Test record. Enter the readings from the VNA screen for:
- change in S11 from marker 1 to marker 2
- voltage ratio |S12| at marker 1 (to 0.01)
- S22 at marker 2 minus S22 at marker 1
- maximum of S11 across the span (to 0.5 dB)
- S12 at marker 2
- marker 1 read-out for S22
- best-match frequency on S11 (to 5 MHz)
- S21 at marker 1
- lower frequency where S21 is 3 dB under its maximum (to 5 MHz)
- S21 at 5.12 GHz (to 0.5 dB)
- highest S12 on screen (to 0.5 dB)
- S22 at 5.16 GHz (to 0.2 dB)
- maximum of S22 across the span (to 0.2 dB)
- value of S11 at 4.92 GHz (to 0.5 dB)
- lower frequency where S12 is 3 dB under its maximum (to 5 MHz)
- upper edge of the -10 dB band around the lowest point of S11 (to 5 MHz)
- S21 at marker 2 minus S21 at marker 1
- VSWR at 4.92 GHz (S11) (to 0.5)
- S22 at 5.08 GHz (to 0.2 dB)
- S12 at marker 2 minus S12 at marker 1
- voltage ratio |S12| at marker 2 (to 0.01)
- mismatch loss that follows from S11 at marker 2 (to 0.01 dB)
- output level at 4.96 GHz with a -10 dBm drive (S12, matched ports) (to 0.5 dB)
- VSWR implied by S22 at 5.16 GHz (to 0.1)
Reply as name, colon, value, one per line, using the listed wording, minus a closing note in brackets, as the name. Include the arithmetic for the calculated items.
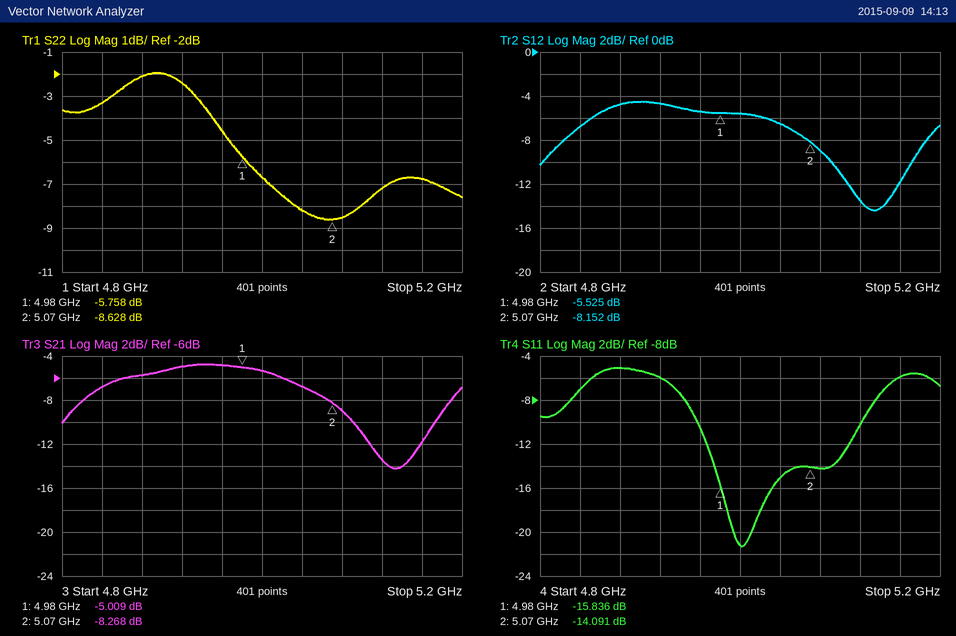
change in S11 from marker 1 to marker 2: -14.091 − (-15.836) = 1.745 dB
voltage ratio |S12| at marker 1: 10^(-5.525/20) ≈ 0.53
S22 at marker 2 minus S22 at marker 1: -8.628 − (-5.758) = -2.870 dB
maximum of S11 across the span: -5.0 dB
S12 at marker 2: -8.152 dB
marker 1 read-out for S22: -5.758 dB
best-match frequency on S11: 5.000 GHz
S21 at marker 1: -5.009 dB
lower frequency where S21 is 3 dB under its maximum: 4.825 GHz
S21 at 5.12 GHz: -13.5 dB
highest S12 on screen: -4.5 dB
S22 at 5.16 GHz: -6.8 dB
maximum of S22 across the span: -2.0 dB
value of S11 at 4.92 GHz: -6.0 dB
lower frequency where S12 is 3 dB under its maximum: 4.830 GHz
upper edge of the -10 dB band around the lowest point of S11: 5.120 GHz
S21 at marker 2 minus S21 at marker 1: -8.268 − (-5.009) = -3.259 dB
VSWR at 4.92 GHz (S11): |Γ| = 10^(-6/20) = 0.5012; VSWR = (1 + 0.5012)/(1 − 0.5012) ≈ 3.0
S22 at 5.08 GHz: -8.6 dB
S12 at marker 2 minus S12 at marker 1: -8.152 − (-5.525) = -2.627 dB
voltage ratio |S12| at marker 2: 10^(-8.152/20) ≈ 0.39
mismatch loss that follows from S11 at marker 2: −10 log10(1 − 10^(-14.091/10)) ≈ 0.17 dB
output level at 4.96 GHz with a -10 dBm drive (S12, matched ports): -10 dBm + (-5.5 dB) = -15.5 dBm
VSWR implied by S22 at 5.16 GHz: |Γ| = 10^(-6.8/20) = 0.4571; VSWR = (1 + 0.4571)/(1 − 0.4571) ≈ 2.7
